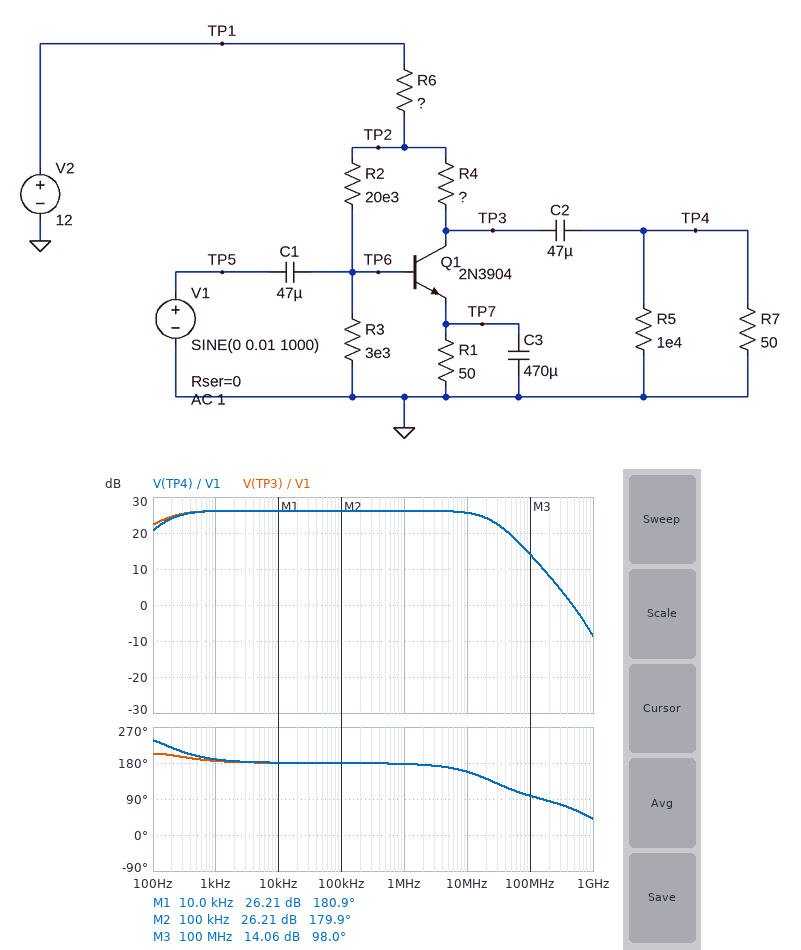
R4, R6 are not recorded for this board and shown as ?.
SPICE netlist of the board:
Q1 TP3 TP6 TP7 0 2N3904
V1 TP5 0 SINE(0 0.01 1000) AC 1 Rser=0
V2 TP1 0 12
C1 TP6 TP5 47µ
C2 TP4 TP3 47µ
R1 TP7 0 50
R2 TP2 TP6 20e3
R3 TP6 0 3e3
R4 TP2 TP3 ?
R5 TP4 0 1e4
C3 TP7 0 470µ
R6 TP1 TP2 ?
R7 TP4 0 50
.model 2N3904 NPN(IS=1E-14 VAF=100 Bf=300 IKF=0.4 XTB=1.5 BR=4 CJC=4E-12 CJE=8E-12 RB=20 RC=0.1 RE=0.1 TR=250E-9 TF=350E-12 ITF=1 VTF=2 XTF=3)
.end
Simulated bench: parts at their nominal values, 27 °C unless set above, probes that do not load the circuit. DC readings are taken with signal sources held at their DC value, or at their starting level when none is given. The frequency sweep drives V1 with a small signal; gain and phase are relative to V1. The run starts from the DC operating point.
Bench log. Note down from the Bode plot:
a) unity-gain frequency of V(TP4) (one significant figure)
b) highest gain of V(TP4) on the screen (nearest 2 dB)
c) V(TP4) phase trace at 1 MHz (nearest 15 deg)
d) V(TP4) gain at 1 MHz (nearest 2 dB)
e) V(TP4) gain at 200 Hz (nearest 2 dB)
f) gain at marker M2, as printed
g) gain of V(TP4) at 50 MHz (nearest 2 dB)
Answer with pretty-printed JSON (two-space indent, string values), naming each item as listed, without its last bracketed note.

{
  "unity-gain frequency of V(TP4)": "500 MHz",
  "highest gain of V(TP4) on the screen": "26 dB",
  "V(TP4) phase trace at 1 MHz": "180 deg",
  "V(TP4) gain at 1 MHz": "26 dB",
  "V(TP4) gain at 200 Hz": "24 dB",
  "gain at marker M2, as printed": "26.21 dB",
  "gain of V(TP4) at 50 MHz": "20 dB"
}
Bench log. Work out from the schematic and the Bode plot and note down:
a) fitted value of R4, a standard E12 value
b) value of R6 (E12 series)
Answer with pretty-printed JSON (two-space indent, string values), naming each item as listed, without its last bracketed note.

{
  "fitted value of R4, a standard E12 value": "820 Ω",
  "value of R6": "56 Ω"
}
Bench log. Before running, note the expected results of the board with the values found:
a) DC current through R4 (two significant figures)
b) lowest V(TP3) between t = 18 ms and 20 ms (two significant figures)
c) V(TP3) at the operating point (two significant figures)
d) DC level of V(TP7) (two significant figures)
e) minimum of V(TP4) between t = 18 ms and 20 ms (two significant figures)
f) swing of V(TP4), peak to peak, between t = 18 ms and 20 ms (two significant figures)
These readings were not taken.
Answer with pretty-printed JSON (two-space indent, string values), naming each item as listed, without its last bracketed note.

{
  "DC current through R4": "13 mA",
  "lowest V(TP3) between t = 18 ms and 20 ms": "760 mV",
  "V(TP3) at the operating point": "930 mV",
  "DC level of V(TP7)": "630 mV",
  "minimum of V(TP4) between t = 18 ms and 20 ms": "-190 mV",
  "swing of V(TP4), peak to peak, between t = 18 ms and 20 ms": "380 mV"
}
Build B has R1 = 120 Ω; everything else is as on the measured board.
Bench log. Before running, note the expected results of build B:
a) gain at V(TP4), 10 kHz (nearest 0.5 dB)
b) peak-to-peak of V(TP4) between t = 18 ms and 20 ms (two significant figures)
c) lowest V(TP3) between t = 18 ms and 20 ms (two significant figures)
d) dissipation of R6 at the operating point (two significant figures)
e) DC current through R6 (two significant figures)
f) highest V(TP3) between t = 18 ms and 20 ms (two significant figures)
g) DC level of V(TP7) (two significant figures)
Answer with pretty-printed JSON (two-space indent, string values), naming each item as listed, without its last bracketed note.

{
  "gain at V(TP4), 10 kHz": "20.5 dB",
  "peak-to-peak of V(TP4) between t = 18 ms and 20 ms": "210 mV",
  "lowest V(TP3) between t = 18 ms and 20 ms": "6.3 V",
  "dissipation of R6 at the operating point": "2.6 mW",
  "DC current through R6": "6.8 mA",
  "highest V(TP3) between t = 18 ms and 20 ms": "6.5 V",
  "DC level of V(TP7)": "760 mV"
}
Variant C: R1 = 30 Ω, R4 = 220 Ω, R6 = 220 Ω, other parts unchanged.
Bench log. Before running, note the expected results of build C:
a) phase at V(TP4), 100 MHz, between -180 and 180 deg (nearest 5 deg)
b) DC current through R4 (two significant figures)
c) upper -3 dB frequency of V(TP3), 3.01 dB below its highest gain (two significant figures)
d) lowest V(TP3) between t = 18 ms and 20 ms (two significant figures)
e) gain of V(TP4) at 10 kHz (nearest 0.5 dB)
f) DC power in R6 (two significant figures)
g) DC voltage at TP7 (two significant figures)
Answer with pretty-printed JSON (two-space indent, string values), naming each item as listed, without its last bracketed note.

{
  "phase at V(TP4), 100 MHz, between -180 and 180 deg": "110 deg",
  "DC current through R4": "12 mA",
  "upper -3 dB frequency of V(TP3), 3.01 dB below its highest gain": "39 MHz",
  "lowest V(TP3) between t = 18 ms and 20 ms": "6.3 V",
  "gain of V(TP4) at 10 kHz": "25.5 dB",
  "DC power in R6": "36 mW",
  "DC voltage at TP7": "370 mV"
}
